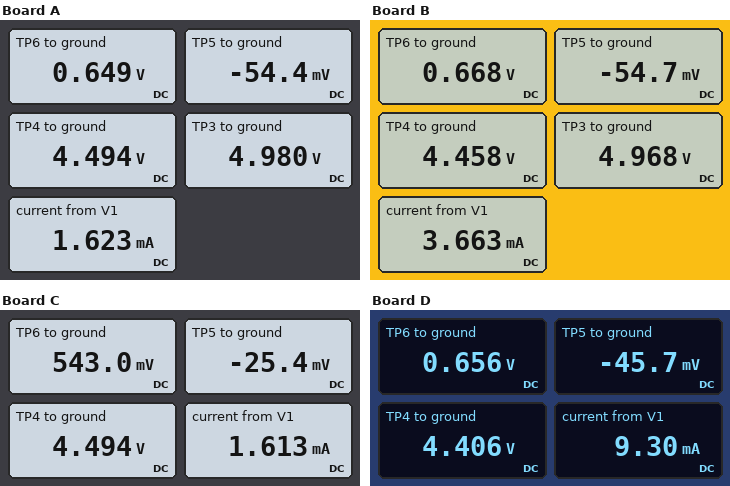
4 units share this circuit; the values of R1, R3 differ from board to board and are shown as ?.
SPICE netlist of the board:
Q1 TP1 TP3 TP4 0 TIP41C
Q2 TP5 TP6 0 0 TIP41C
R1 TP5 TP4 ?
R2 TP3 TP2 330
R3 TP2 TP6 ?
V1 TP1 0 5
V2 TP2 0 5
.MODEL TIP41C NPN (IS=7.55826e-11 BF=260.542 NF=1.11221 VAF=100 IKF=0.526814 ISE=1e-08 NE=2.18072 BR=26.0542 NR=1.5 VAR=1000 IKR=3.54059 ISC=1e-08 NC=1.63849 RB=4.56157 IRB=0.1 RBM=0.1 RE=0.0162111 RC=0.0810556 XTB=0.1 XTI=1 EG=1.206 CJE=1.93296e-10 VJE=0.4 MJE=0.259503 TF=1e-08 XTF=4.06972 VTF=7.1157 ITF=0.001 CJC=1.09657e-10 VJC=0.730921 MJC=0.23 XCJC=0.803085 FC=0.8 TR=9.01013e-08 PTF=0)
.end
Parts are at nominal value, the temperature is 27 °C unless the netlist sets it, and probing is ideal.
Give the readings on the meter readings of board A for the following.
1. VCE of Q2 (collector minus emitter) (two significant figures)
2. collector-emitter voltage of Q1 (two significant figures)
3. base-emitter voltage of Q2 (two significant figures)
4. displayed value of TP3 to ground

-54 mV
510 mV
650 mV
4.980 V
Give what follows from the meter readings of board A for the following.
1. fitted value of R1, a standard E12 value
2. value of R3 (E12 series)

2.7 kΩ
180 Ω
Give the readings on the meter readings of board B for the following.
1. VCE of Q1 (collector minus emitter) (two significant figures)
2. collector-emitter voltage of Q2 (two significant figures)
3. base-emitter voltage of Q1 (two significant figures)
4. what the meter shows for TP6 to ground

540 mV
-55 mV
510 mV
0.668 V
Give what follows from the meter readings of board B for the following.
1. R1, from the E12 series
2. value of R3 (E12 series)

1.2 kΩ
150 Ω
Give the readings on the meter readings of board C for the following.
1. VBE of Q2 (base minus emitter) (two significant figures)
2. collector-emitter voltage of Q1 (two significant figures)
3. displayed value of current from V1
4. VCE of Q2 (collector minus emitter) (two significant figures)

540 mV
510 mV
1.613 mA
-25 mV
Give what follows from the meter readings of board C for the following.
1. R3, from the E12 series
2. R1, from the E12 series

1 kΩ
2.7 kΩ
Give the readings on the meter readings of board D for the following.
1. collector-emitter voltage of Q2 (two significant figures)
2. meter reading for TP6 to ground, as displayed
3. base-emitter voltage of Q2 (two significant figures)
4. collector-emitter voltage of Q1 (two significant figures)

-46 mV
0.656 V
660 mV
590 mV
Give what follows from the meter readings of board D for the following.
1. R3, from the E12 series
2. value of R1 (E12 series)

180 Ω
470 Ω
